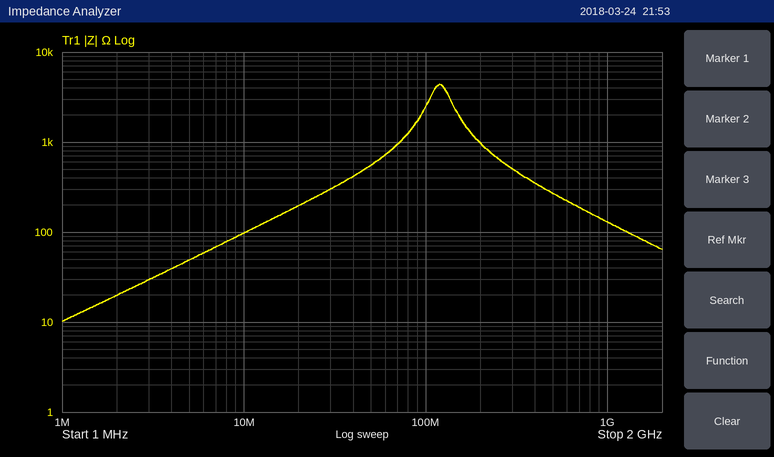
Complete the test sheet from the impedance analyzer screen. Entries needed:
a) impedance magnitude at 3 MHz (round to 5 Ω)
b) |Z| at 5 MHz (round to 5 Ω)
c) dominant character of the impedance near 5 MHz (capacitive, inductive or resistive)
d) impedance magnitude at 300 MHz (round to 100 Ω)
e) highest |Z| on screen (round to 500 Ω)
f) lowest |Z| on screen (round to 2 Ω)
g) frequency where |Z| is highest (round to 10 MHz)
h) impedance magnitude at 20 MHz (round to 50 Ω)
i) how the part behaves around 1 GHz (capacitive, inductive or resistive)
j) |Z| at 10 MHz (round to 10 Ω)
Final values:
30 Ω
50 Ω
inductive
500 Ω
4.5 kΩ
10 Ω
120 MHz
200 Ω
capacitive
100 Ω
